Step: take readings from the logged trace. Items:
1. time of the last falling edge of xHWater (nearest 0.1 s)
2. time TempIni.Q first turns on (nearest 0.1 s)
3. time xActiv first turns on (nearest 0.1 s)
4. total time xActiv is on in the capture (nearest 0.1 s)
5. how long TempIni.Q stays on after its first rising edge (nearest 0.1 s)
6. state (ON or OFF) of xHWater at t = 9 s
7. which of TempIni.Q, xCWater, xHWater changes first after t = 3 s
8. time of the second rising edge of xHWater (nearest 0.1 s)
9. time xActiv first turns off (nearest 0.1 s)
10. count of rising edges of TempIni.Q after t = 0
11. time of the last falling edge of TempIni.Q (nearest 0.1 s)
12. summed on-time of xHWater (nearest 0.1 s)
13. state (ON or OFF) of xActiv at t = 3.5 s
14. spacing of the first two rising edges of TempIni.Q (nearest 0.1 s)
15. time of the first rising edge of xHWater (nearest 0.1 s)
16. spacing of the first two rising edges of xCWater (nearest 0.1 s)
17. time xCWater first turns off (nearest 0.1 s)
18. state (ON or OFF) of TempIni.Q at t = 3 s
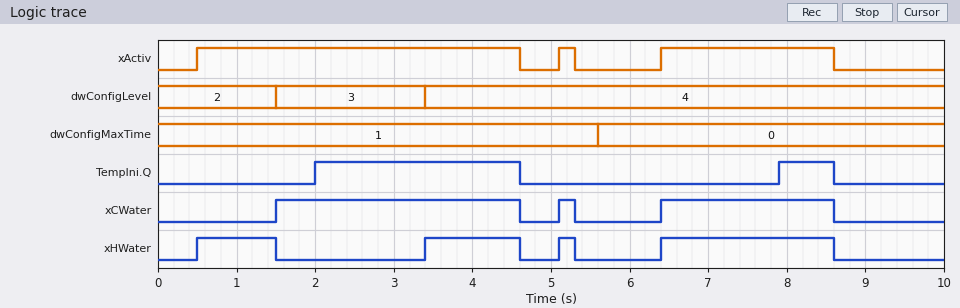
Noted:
8.6 s
2.0 s
0.5 s
6.5 s
2.6 s
OFF
xHWater
3.4 s
4.6 s
2
8.6 s
4.6 s
ON
5.9 s
0.5 s
3.6 s
4.6 s
ON
